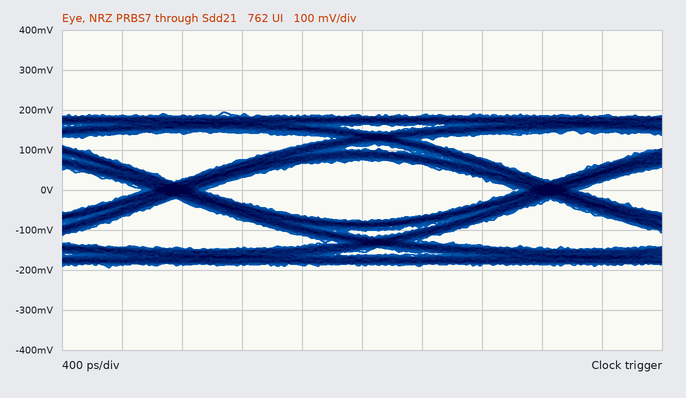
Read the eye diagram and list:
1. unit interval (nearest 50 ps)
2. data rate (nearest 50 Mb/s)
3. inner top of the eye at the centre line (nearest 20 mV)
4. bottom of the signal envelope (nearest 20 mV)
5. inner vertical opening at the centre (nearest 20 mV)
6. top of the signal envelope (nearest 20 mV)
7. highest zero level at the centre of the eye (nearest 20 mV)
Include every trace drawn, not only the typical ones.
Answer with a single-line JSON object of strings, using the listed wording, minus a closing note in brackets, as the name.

{"unit interval": "2.50 ns", "data rate": "400 Mb/s", "inner top of the eye at the centre line": "80 mV", "bottom of the signal envelope": "-200 mV", "inner vertical opening at the centre": "160 mV", "top of the signal envelope": "200 mV", "highest zero level at the centre of the eye": "-80 mV"}
